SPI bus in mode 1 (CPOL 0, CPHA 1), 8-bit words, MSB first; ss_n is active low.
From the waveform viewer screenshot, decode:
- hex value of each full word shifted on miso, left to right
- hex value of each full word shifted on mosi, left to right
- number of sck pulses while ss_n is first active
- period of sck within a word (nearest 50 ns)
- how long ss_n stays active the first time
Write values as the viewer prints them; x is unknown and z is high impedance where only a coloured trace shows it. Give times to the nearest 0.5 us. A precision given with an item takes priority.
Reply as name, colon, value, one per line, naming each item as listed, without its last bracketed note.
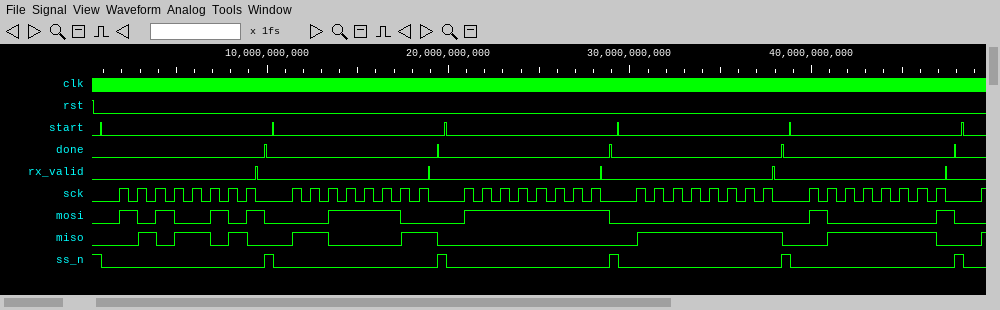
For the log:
hex value of each full word shifted on miso, left to right: 5A, C3, 00, FF, 7E
hex value of each full word shifted on mosi, left to right: A5, 3C, FF, 00, 81
number of sck pulses while ss_n is first active: 8
period of sck within a word: 1000 ns
how long ss_n stays active the first time: 9 us
